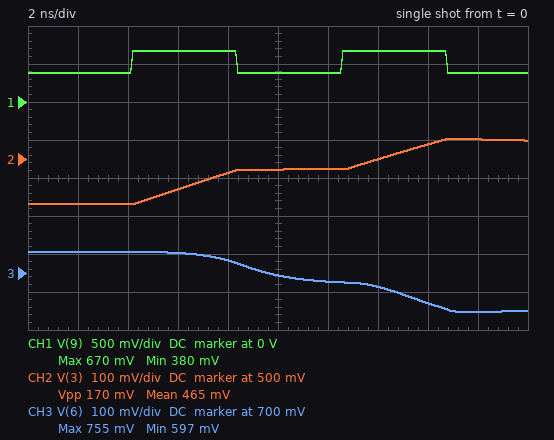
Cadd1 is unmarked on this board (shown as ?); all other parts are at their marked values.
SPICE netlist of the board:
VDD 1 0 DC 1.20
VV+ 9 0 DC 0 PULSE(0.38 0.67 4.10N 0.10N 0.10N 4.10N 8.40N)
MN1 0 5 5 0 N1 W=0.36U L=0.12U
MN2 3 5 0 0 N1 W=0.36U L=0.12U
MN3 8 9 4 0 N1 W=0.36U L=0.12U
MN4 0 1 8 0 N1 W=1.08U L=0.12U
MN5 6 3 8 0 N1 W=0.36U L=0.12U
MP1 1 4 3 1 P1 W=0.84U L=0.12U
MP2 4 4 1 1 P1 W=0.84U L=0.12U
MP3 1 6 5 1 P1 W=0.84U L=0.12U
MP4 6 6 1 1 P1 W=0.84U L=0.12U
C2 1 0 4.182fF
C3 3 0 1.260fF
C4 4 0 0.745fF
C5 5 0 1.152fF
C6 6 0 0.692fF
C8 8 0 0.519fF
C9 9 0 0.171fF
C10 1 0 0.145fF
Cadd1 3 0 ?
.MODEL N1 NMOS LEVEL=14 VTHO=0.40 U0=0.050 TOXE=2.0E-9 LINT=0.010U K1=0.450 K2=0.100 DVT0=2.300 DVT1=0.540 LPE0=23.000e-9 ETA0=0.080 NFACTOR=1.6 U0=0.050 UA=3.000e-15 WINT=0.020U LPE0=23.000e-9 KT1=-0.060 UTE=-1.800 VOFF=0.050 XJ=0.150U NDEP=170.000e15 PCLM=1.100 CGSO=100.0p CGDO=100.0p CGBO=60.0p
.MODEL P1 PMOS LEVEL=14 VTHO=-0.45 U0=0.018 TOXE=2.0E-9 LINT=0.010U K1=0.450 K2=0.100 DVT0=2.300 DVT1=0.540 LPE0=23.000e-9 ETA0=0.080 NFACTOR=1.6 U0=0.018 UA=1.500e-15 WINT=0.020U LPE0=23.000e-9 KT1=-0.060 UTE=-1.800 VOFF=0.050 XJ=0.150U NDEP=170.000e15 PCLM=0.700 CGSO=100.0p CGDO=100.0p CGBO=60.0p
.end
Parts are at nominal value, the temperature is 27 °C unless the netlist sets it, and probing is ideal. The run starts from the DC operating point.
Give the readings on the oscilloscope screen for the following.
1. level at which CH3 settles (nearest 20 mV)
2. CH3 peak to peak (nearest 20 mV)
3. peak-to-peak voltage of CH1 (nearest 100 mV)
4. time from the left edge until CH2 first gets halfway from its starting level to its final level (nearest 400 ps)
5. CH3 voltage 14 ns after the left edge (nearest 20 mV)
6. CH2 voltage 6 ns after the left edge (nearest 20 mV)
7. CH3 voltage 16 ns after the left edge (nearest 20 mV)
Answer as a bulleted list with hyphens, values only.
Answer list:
- 600 mV
- 160 mV
- 300 mV
- 8.0 ns
- 660 mV
- 420 mV
- 620 mV
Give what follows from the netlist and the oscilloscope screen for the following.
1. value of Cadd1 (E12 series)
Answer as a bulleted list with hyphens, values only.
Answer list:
- 390 fF
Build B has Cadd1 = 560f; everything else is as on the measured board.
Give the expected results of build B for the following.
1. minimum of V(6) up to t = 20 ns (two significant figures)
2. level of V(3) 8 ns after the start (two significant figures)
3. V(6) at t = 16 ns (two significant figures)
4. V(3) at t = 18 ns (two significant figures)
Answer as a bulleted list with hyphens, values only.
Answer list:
- 640 mV
- 440 mV
- 670 mV
- 510 mV
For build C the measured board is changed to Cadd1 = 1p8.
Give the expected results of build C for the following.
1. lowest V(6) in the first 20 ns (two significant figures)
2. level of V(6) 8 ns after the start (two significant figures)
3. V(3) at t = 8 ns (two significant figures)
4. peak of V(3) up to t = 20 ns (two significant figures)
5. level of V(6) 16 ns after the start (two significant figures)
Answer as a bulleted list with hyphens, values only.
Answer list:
- 730 mV
- 750 mV
- 400 mV
- 420 mV
- 740 mV
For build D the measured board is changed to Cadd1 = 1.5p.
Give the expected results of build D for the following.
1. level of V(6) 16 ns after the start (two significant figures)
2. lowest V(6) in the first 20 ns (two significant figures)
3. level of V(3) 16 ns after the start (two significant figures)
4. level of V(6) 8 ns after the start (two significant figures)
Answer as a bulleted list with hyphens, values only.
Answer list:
- 740 mV
- 720 mV
- 430 mV
- 750 mV
